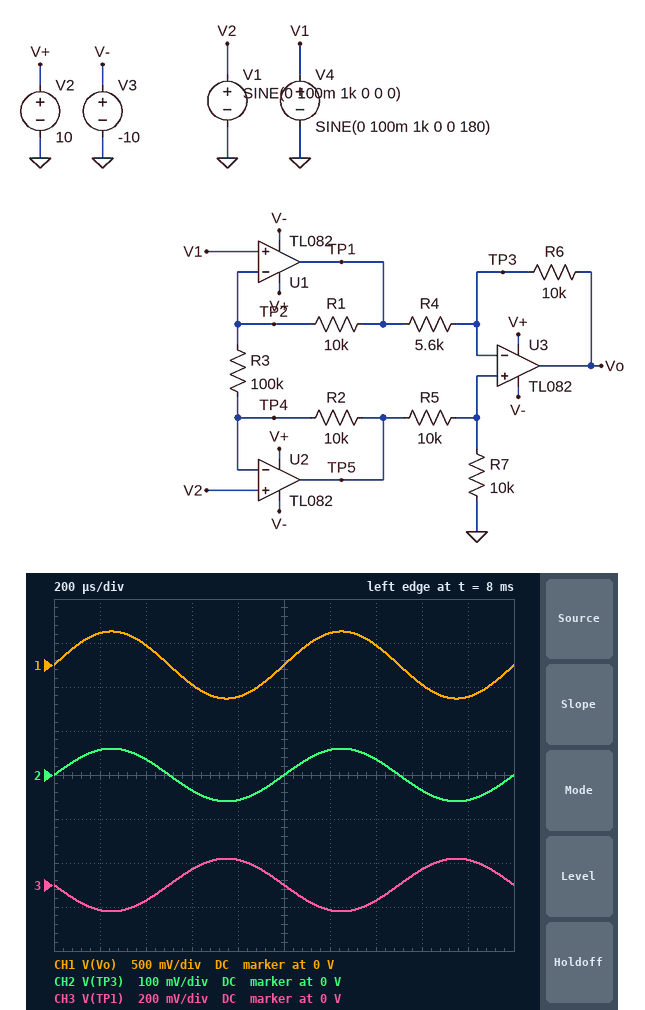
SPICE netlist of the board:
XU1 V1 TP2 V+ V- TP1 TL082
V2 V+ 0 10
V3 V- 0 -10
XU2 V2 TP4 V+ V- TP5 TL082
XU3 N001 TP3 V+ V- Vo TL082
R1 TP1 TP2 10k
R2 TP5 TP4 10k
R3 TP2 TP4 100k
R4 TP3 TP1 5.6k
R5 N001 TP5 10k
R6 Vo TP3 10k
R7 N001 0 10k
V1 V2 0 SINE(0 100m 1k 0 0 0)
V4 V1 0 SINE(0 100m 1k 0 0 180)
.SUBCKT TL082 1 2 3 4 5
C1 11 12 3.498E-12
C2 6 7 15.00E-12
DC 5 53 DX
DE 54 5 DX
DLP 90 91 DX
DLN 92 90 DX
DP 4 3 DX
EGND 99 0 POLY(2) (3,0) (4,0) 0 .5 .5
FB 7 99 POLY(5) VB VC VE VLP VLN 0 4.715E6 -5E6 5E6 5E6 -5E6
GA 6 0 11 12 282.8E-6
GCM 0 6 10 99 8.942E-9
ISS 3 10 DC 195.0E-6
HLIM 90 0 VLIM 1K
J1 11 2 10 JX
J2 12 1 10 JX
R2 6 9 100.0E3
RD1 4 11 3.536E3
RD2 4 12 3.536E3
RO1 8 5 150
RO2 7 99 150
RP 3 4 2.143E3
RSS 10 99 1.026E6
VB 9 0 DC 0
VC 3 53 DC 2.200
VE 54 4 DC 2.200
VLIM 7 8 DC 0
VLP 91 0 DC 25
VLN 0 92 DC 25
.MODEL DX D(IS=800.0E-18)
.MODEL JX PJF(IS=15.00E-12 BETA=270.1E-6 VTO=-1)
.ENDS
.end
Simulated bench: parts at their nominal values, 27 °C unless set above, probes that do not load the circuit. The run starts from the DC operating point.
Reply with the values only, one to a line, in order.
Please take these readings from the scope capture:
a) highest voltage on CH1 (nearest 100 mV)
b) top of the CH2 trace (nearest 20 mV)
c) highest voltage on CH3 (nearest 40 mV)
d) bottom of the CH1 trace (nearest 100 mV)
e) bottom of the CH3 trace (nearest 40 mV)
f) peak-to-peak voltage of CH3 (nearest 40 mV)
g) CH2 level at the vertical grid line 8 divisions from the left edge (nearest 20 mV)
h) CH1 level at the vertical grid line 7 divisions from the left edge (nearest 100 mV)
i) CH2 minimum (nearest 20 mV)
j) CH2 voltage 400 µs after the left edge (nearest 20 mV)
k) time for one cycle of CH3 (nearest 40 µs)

400 mV
60 mV
120 mV
-400 mV
-120 mV
240 mV
-40 mV
200 mV
-60 mV
40 mV
1.00 ms
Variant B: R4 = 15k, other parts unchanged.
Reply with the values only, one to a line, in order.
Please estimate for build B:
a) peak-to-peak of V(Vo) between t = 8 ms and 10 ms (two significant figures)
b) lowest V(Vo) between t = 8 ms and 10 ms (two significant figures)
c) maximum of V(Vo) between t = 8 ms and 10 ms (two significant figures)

360 mV
-180 mV
180 mV
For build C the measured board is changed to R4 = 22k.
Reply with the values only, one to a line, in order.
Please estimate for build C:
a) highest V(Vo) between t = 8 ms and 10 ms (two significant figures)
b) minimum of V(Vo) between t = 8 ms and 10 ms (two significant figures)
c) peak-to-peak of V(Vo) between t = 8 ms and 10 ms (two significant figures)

140 mV
-140 mV
280 mV
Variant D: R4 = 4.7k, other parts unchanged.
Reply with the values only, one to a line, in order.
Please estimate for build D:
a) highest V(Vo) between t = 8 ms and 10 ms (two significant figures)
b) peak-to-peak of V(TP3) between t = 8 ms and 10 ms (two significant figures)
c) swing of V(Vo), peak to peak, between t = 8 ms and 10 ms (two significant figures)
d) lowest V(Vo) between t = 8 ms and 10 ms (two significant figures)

440 mV
120 mV
890 mV
-440 mV
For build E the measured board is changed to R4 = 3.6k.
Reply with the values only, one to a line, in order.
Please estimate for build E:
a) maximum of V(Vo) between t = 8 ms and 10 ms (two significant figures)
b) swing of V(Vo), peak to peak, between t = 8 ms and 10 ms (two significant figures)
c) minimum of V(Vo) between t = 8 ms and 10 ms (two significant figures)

560 mV
1.1 V
-560 mV
